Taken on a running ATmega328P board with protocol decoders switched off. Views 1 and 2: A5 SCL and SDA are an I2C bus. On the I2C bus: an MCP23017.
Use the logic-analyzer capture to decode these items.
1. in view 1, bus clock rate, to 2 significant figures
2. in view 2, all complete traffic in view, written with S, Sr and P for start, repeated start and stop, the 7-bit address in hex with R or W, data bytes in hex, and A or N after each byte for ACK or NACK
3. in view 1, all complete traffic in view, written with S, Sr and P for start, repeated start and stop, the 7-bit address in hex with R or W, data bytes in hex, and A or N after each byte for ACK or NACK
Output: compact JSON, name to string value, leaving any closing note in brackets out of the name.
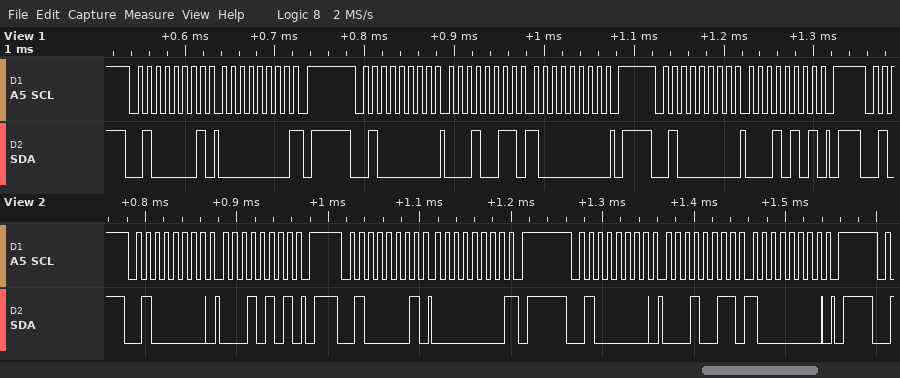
{"in view 1, bus clock rate, to 2 significant figures": "100 kHz", "in view 2, all complete traffic in view, written with S, Sr and P for start, repeated start and stop, the 7-bit address in hex with R or W, data bytes in hex, and A or N after each byte for ACK or NACK": "S 20W A 15 A P S 20R A 00 N P S 20W A 13 A 80 A P", "in view 1, all complete traffic in view, written with S, Sr and P for start, repeated start and stop, the 7-bit address in hex with R or W, data bytes in hex, and A or N after each byte for ACK or NACK": "S 20R A 00 N P S 20W A 13 A 80 A P S 20W A 15 A P"}
